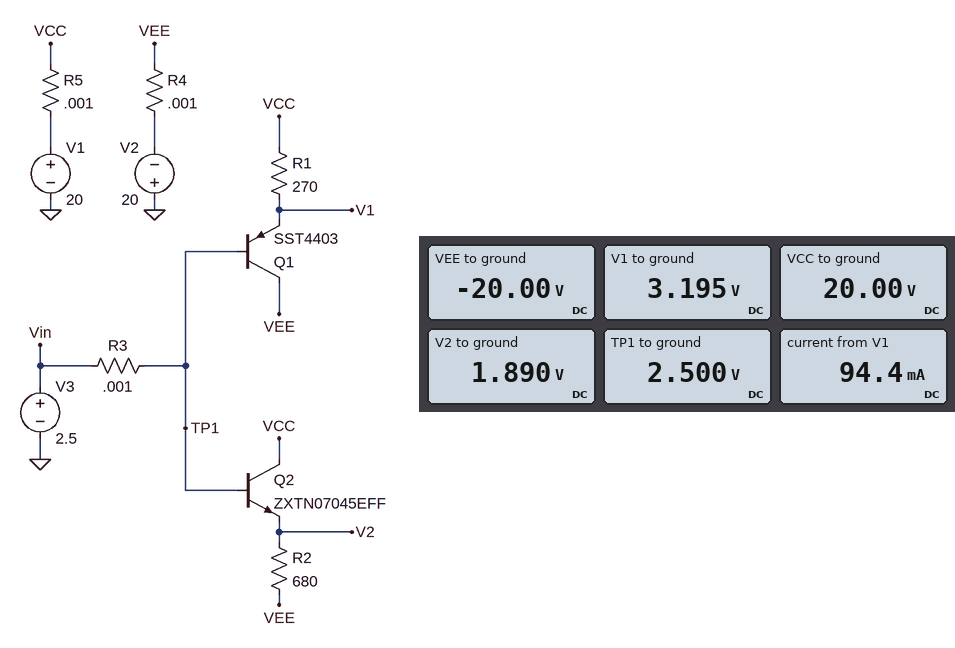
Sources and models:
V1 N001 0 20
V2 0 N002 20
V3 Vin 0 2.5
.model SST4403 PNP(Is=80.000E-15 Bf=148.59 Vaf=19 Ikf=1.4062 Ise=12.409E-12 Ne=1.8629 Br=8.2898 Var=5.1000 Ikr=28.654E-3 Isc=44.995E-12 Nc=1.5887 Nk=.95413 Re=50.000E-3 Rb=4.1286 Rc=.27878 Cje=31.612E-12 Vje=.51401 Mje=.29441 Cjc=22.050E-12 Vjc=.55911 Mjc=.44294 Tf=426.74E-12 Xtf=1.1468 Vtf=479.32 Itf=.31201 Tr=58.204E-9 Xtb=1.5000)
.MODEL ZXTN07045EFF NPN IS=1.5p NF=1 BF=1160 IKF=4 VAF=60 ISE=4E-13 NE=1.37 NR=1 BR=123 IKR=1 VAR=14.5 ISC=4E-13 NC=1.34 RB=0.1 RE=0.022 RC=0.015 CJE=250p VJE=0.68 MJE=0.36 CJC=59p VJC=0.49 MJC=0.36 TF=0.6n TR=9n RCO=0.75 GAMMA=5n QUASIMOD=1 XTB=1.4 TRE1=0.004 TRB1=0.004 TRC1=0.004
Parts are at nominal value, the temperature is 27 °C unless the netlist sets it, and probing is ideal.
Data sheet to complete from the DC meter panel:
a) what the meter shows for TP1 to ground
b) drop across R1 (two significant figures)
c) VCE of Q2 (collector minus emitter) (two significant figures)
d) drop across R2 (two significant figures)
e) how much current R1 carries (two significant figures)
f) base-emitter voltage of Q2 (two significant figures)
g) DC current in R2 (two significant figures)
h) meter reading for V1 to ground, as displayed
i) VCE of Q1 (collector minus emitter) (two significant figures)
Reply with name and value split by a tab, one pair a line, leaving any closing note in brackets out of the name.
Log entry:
what the meter shows for TP1 to ground	2.500 V
drop across R1	17 V
VCE of Q2 (collector minus emitter)	18 V
drop across R2	22 V
how much current R1 carries	62 mA
base-emitter voltage of Q2	610 mV
DC current in R2	32 mA
meter reading for V1 to ground, as displayed	3.195 V
VCE of Q1 (collector minus emitter)	-23 V
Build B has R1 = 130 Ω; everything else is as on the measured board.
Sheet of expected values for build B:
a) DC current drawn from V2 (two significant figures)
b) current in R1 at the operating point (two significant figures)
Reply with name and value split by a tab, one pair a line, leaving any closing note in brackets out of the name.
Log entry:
DC current drawn from V2	160 mA
current in R1 at the operating point	130 mA
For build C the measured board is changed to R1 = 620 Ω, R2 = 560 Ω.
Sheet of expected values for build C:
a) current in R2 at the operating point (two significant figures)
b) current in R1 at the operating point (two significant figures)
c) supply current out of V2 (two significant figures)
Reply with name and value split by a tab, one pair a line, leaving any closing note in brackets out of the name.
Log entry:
current in R2 at the operating point	39 mA
current in R1 at the operating point	27 mA
supply current out of V2	66 mA
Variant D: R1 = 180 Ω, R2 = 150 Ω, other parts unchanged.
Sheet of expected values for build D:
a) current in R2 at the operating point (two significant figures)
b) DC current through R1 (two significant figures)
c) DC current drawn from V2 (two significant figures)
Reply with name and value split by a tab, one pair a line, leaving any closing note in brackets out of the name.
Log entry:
current in R2 at the operating point	150 mA
DC current through R1	93 mA
DC current drawn from V2	240 mA
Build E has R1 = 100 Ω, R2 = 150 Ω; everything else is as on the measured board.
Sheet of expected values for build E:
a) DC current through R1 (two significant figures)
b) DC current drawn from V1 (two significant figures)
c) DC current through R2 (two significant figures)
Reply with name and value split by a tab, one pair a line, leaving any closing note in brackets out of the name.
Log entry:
DC current through R1	170 mA
DC current drawn from V1	310 mA
DC current through R2	150 mA
